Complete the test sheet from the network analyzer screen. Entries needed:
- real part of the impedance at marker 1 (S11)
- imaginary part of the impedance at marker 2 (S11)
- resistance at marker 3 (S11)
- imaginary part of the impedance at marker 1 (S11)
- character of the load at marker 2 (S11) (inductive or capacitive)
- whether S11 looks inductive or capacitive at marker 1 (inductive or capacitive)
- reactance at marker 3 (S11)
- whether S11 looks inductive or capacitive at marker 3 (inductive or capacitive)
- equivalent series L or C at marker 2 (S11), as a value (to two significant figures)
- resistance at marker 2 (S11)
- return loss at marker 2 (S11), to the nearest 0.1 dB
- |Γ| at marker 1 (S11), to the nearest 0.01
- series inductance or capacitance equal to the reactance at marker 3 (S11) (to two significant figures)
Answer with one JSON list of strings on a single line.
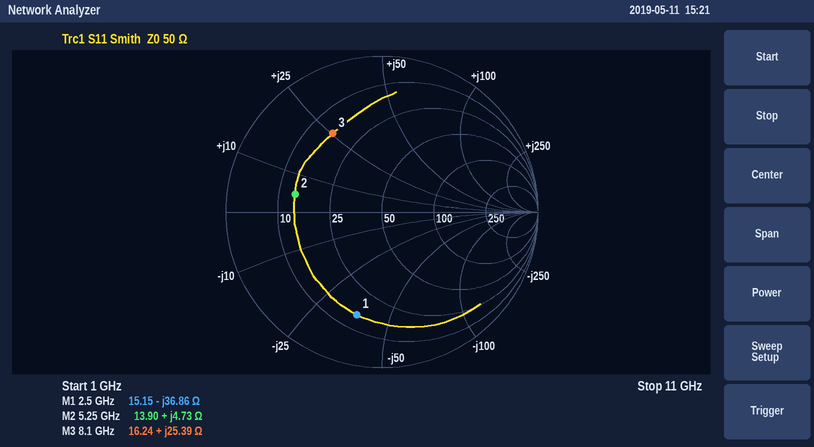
["15.15 Ω", "+4.73 Ω", "16.24 Ω", "-36.86 Ω", "inductive", "capacitive", "+25.39 Ω", "inductive", "140 pH", "13.90 Ω", "4.9 dB", "0.68", "500 pH"]
